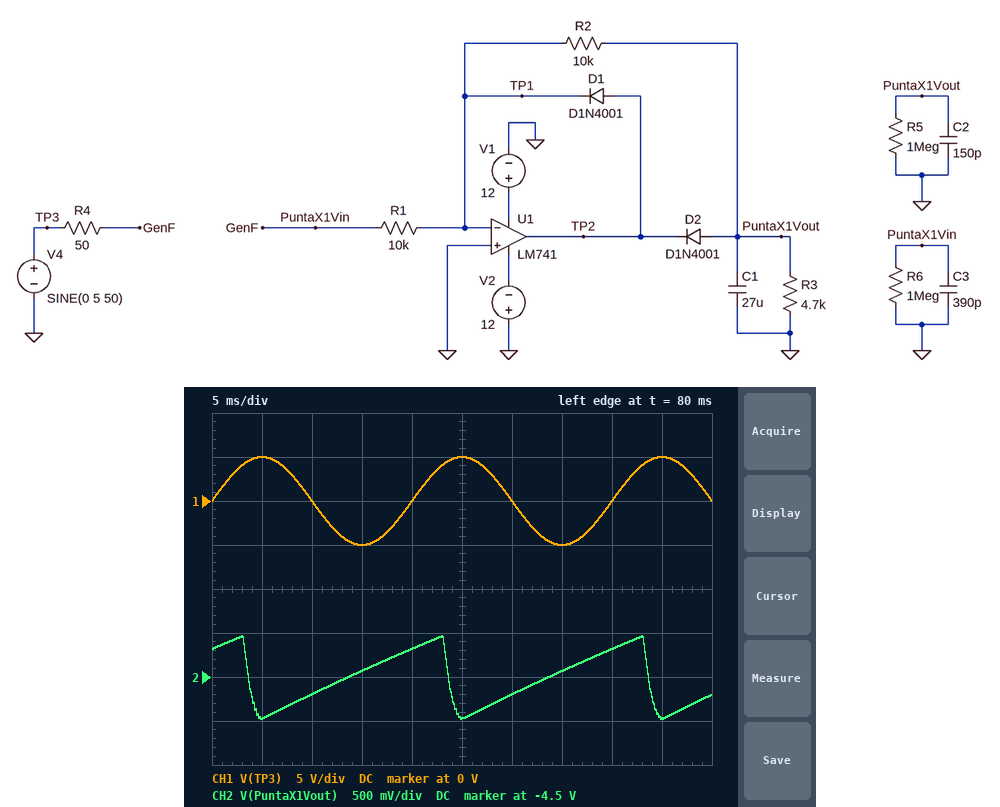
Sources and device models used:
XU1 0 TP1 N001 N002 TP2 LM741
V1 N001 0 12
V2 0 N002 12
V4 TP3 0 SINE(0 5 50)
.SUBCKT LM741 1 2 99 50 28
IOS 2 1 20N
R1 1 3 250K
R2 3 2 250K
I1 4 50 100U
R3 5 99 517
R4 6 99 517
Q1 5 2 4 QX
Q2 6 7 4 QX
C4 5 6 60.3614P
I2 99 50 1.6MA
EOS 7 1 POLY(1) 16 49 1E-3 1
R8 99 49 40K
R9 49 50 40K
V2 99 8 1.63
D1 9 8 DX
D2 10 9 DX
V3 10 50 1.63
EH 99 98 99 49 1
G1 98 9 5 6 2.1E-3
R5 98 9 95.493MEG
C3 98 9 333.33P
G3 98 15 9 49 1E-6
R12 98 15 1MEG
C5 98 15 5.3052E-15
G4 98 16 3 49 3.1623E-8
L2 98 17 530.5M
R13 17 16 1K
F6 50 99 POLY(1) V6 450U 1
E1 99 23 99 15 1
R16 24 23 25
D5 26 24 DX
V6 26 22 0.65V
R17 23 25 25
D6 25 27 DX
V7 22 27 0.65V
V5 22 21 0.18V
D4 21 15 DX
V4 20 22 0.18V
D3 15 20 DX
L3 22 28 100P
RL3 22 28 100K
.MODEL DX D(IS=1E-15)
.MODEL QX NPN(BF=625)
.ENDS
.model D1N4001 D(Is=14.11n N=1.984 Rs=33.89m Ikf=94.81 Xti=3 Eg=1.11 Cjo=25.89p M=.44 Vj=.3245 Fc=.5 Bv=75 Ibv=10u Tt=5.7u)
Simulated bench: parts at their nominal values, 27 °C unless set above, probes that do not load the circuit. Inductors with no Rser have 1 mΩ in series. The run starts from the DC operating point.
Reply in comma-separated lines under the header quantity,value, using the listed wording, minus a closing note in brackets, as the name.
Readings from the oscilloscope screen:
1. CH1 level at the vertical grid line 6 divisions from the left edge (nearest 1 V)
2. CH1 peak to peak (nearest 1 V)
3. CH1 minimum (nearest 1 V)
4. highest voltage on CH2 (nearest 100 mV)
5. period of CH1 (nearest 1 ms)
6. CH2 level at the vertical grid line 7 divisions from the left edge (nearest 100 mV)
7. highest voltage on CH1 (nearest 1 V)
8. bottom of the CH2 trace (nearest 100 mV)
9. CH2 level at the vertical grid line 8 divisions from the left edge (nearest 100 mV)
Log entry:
quantity,value
CH1 level at the vertical grid line 6 divisions from the left edge,0 V
CH1 peak to peak,10 V
CH1 minimum,-5 V
highest voltage on CH2,-4.0 V
period of CH1,20 ms
CH2 level at the vertical grid line 7 divisions from the left edge,-4.4 V
highest voltage on CH1,5 V
bottom of the CH2 trace,-5.0 V
CH2 level at the vertical grid line 8 divisions from the left edge,-4.2 V
